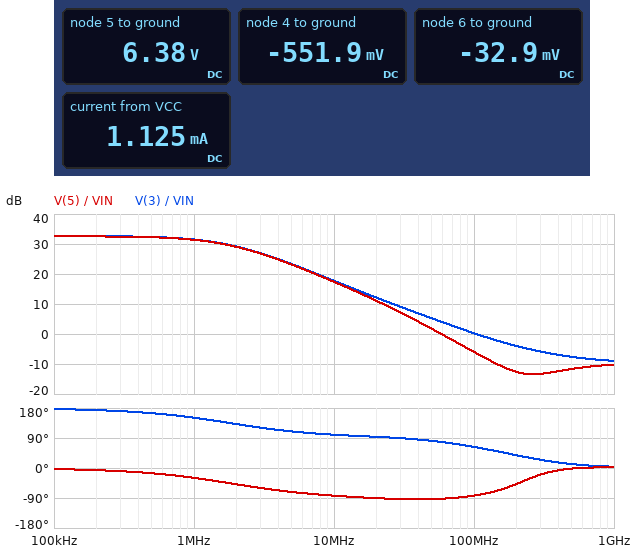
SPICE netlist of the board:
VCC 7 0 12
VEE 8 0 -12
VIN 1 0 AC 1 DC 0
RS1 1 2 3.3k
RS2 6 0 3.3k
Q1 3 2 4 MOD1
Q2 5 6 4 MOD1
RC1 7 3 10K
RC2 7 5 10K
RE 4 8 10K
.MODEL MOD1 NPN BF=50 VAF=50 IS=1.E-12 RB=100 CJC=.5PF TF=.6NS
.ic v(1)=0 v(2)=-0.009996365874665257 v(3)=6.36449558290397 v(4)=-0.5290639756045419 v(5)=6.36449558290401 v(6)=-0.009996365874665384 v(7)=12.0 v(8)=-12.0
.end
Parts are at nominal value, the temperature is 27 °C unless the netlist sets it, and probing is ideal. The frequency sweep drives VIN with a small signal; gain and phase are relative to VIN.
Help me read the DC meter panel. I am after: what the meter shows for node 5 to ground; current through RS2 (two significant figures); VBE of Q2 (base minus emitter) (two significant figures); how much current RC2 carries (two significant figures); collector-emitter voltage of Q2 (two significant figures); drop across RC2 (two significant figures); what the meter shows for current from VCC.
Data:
6.38 V
10 µA
520 mV
560 µA
6.9 V
5.6 V
1.125 mA
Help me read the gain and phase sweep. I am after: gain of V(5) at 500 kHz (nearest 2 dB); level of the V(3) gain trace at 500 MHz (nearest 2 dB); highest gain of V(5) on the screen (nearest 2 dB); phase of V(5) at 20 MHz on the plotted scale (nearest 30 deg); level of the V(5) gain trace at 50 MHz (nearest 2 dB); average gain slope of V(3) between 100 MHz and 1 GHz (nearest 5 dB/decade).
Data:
32 dB
-8 dB
32 dB
-90 deg
2 dB
-10 dB/decade
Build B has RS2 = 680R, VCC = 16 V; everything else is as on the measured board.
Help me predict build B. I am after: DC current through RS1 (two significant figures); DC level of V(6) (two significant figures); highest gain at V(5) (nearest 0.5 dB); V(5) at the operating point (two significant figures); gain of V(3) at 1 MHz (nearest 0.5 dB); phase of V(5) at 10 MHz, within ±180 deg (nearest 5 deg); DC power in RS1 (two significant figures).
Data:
6.9 µA
-8.1 mV
35.0 dB
9.0 V
34.5 dB
-80 deg
160 nW
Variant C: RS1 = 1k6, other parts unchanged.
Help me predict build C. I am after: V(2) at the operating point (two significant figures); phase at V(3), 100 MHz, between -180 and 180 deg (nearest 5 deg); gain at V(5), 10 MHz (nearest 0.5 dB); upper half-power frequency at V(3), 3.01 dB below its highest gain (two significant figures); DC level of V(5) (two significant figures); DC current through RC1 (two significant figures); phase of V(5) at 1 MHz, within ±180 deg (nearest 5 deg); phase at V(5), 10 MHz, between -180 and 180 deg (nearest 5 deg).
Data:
-19 mV
65 deg
20.0 dB
2.1 MHz
7.2 V
650 µA
-25 deg
-80 deg
